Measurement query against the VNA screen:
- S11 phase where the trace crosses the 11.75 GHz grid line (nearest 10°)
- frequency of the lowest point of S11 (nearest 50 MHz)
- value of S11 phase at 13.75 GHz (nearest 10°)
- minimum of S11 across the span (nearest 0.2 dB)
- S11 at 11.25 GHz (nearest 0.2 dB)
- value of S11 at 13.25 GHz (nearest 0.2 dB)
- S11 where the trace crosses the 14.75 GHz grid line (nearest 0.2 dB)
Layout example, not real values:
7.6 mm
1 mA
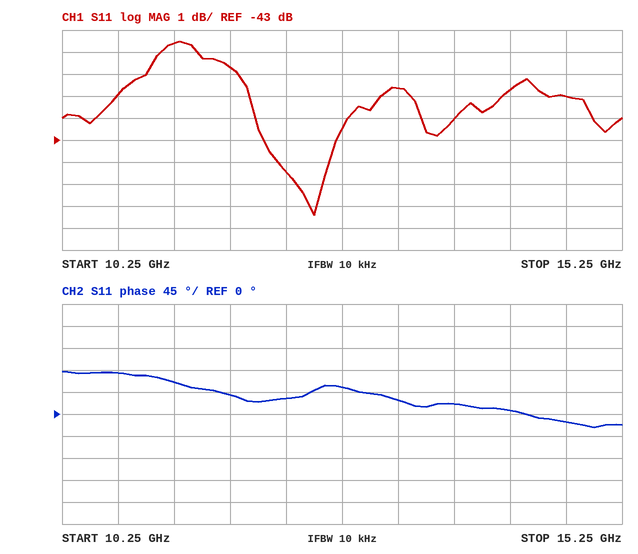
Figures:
40°
12.50 GHz
20°
-46.4 dB
-38.6 dB
-40.6 dB
-41.0 dB
